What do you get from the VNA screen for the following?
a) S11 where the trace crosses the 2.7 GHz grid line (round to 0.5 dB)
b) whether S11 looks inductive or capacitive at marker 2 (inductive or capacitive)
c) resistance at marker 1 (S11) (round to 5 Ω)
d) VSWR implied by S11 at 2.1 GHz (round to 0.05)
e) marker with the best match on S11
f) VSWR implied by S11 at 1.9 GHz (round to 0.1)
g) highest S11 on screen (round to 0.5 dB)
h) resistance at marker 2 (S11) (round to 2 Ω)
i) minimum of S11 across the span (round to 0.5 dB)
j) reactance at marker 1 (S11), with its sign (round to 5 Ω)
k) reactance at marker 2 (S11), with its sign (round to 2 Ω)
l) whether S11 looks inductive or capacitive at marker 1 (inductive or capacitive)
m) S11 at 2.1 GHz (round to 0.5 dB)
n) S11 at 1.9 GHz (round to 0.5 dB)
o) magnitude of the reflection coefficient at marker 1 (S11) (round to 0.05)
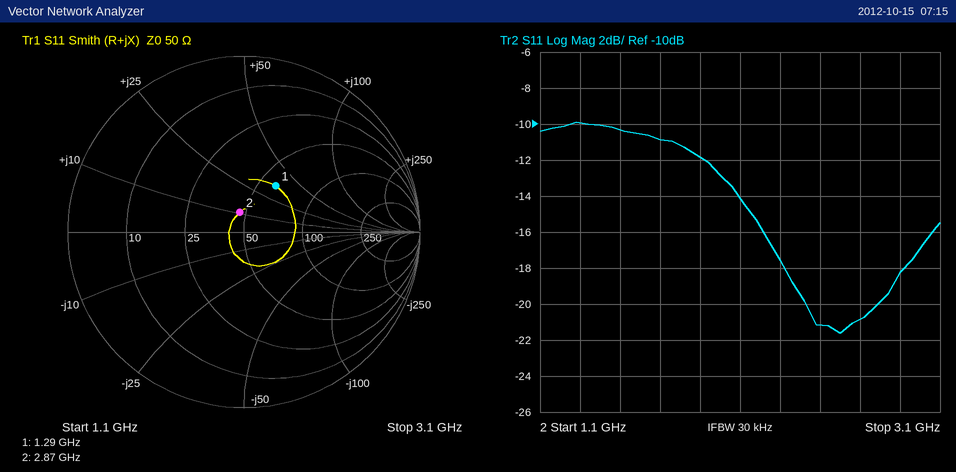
-21.0 dB
inductive
60 Ω
1.50
marker 2
1.7
-10.0 dB
46 Ω
-21.5 dB
+35 Ω
+10 Ω
inductive
-14.0 dB
-12.0 dB
0.30
